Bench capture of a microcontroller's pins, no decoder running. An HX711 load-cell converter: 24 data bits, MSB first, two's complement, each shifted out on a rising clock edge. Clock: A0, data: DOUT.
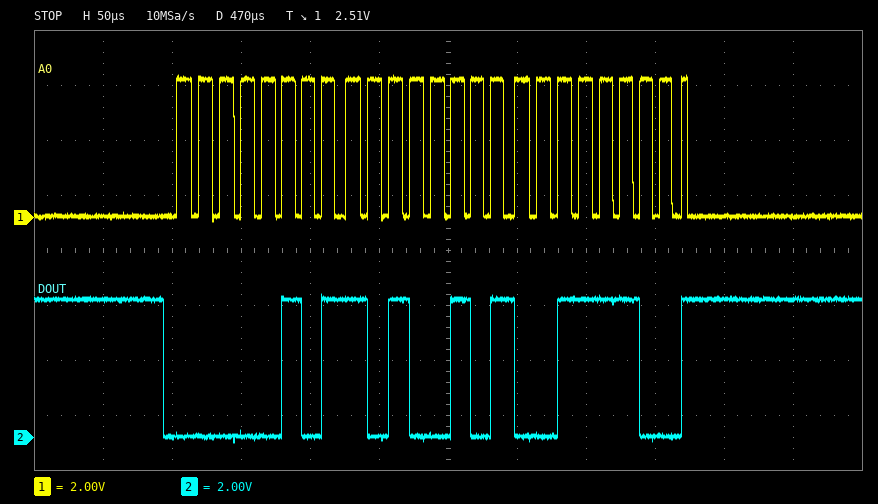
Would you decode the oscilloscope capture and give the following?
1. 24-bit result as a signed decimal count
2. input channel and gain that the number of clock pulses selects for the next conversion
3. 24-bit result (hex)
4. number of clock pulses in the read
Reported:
369980
channel A, gain 128
0x05A53C
25
